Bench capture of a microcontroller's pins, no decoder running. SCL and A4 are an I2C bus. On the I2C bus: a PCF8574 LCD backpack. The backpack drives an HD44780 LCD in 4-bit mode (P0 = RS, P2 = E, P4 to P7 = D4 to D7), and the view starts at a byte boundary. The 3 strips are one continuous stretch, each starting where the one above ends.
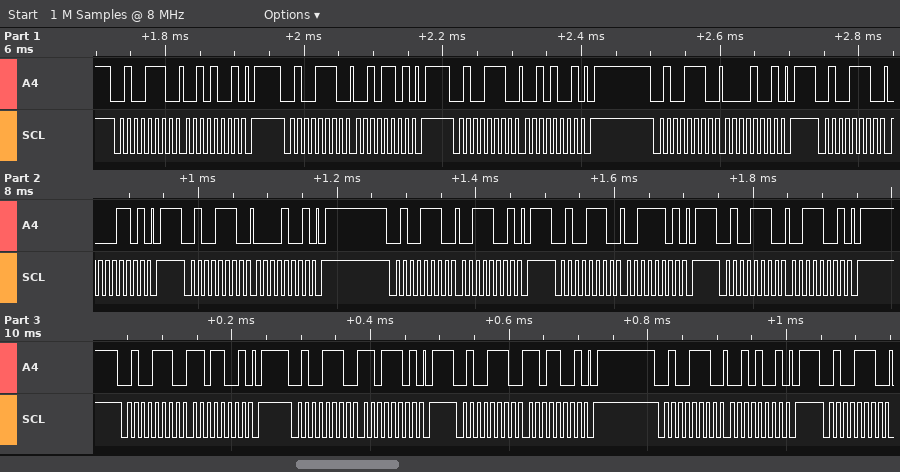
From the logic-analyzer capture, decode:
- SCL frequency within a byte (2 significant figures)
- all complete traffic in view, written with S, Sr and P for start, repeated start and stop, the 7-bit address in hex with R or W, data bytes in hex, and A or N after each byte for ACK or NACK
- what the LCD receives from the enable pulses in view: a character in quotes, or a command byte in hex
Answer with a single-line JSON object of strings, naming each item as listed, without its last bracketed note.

{"SCL frequency within a byte": "100 kHz", "all complete traffic in view, written with S, Sr and P for start, repeated start and stop, the 7-bit address in hex with R or W, data bytes in hex, and A or N after each byte for ACK or NACK": "S 27W A 29 A P S 27W A 2D A P S 27W A 29 A P S 27W A 09 A P S 27W A 0D A P S 27W A 09 A P S 27W A 39 A P S 27W A 3D A P S 27W A 39 A P S 27W A D9 A P S 27W A DD A P S 27W A D9 A P S 27W A 29 A P S 27W A", "what the LCD receives from the enable pulses in view: a character in quotes, or a command byte in hex": "' ' '='"}
